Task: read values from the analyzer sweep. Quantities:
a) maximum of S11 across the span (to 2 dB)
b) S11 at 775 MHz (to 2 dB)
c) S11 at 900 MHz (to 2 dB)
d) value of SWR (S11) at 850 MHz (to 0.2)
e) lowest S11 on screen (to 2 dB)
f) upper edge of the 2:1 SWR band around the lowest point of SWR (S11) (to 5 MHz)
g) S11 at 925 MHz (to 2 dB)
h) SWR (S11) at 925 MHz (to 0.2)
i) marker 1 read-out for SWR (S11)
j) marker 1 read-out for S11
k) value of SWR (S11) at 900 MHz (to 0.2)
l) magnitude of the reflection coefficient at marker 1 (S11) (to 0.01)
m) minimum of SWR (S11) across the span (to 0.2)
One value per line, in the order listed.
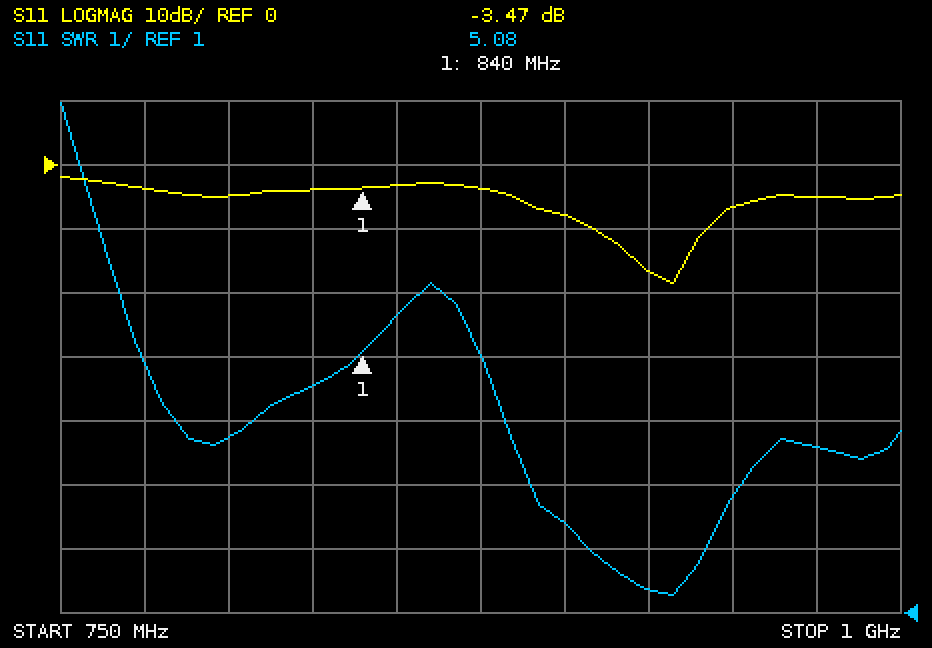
-2 dB
-4 dB
-8 dB
5.6
-18 dB
940 MHz
-16 dB
1.4
5.08
-3.47 dB
2.4
0.67
1.2
